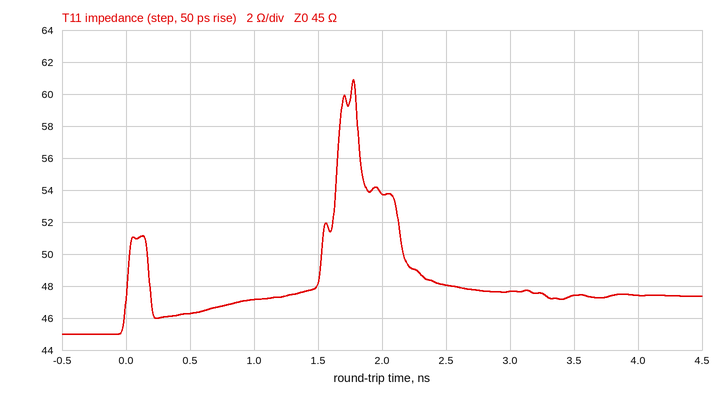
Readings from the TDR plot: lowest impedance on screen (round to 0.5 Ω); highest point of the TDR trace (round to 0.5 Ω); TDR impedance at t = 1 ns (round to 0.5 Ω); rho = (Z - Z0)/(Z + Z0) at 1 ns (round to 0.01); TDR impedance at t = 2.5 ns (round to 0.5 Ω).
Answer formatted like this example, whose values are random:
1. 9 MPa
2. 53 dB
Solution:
1. 45.0 Ω
2. 61.0 Ω
3. 47.0 Ω
4. +0.02
5. 48.0 Ω
